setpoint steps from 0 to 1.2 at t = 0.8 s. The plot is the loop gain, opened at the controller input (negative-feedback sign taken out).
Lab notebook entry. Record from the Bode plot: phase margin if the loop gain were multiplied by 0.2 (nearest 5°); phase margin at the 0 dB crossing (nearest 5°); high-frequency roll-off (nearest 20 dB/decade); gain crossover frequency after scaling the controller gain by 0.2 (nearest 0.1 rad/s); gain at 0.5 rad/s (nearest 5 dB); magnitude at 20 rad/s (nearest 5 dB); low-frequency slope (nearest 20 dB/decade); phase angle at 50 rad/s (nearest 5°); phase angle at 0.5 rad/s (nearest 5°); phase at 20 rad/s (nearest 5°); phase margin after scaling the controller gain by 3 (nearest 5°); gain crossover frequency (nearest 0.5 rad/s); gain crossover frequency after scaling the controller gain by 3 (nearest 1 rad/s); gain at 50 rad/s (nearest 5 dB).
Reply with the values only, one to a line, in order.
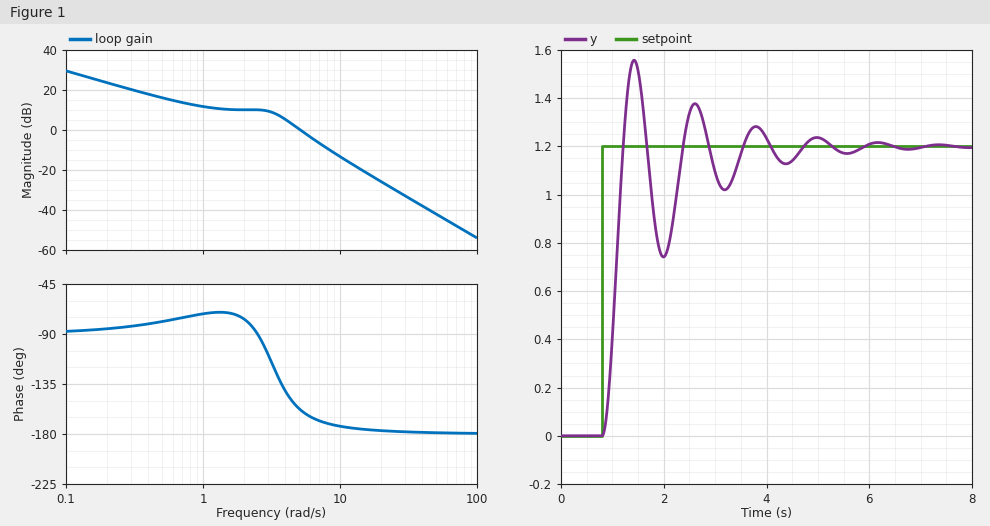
105°
20°
-40 dB/decade
0.7 rad/s
15 dB
-25 dB
-20 dB/decade
-180°
-80°
-175°
10°
5.0 rad/s
8 rad/s
-40 dB
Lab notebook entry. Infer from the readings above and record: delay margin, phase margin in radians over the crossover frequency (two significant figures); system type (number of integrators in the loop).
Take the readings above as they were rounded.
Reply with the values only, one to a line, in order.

0.070 s
1
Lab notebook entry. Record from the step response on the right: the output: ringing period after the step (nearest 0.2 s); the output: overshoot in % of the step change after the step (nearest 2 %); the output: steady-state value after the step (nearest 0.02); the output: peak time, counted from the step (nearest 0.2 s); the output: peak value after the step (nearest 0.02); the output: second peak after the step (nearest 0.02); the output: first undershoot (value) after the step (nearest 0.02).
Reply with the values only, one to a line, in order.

1.2 s
30 %
1.20
0.6 s
1.56
1.38
0.74
